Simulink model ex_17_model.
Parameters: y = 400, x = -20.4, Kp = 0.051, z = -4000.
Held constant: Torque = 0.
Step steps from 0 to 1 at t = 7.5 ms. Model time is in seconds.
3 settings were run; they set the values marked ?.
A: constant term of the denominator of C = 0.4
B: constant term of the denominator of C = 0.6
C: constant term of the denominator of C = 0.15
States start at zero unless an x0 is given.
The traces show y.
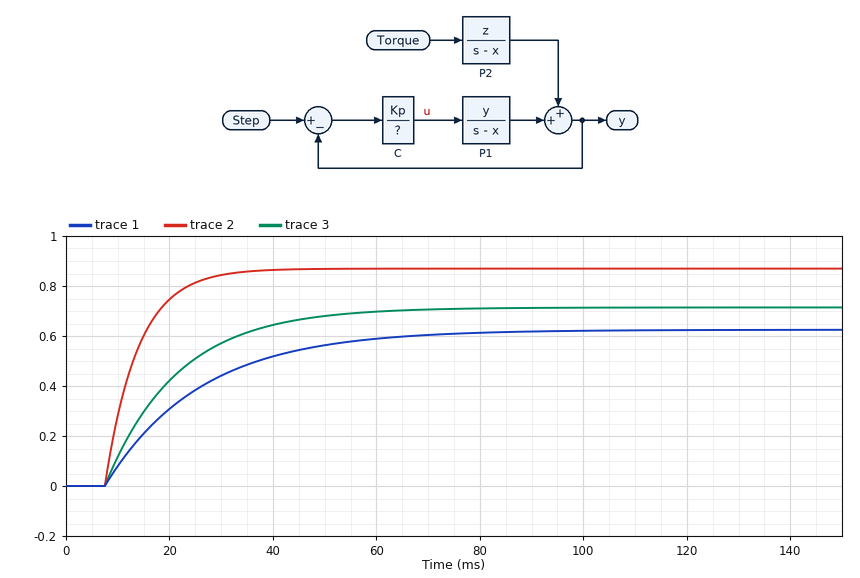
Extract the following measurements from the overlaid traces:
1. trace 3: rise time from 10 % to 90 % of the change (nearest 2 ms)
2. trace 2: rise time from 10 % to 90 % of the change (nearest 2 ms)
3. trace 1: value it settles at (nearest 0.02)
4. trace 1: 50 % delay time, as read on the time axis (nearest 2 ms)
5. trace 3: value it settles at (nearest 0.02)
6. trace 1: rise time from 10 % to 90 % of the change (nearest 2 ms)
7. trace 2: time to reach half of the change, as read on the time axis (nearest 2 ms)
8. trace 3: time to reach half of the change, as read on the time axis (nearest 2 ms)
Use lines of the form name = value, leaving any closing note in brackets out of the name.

trace 3: rise time from 10 % to 90 % of the change = 30 ms
trace 2: rise time from 10 % to 90 % of the change = 14 ms
trace 1: value it settles at = 0.62
trace 1: 50 % delay time, as read on the time axis = 20 ms
trace 3: value it settles at = 0.72
trace 1: rise time from 10 % to 90 % of the change = 40 ms
trace 2: time to reach half of the change, as read on the time axis = 12 ms
trace 3: time to reach half of the change, as read on the time axis = 18 ms
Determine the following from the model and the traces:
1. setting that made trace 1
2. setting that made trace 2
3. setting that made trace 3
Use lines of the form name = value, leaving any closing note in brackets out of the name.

setting that made trace 1 = B
setting that made trace 2 = C
setting that made trace 3 = A
